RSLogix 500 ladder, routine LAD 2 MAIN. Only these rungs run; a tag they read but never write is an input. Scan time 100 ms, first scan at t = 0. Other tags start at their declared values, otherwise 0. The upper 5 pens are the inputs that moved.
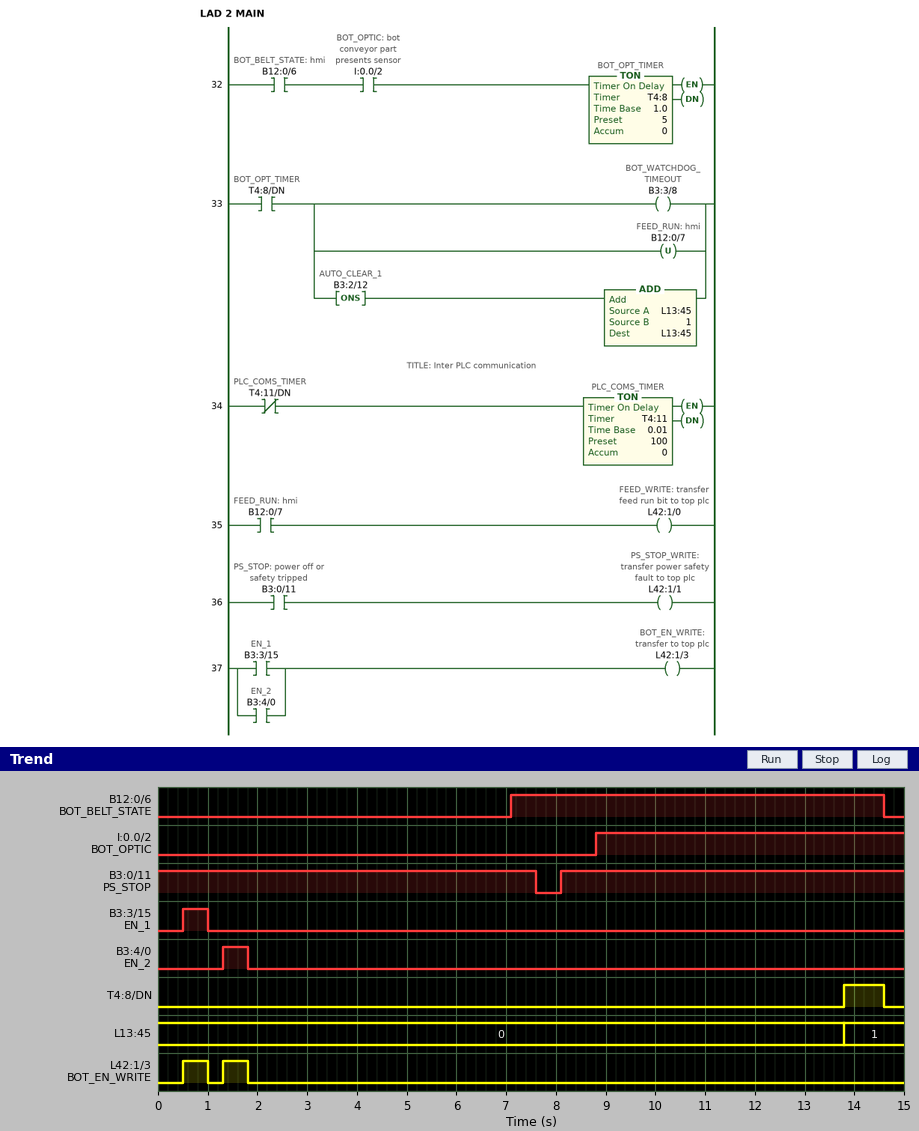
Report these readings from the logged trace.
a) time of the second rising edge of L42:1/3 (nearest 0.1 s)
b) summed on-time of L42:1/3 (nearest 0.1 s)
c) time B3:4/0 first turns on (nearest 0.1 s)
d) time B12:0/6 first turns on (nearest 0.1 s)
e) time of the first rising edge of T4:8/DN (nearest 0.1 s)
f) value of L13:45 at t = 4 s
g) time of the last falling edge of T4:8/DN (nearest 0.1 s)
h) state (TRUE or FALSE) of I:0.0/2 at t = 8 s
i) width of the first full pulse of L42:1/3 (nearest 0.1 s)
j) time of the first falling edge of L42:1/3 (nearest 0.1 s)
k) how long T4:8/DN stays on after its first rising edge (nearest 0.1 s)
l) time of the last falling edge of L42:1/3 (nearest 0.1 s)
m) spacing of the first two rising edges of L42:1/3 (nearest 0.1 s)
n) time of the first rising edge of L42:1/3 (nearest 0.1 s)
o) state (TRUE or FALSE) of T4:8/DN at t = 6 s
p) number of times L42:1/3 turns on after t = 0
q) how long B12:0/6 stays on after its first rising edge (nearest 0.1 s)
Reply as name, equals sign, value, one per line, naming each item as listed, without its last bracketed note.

time of the second rising edge of L42:1/3 = 1.3 s
summed on-time of L42:1/3 = 1.0 s
time B3:4/0 first turns on = 1.3 s
time B12:0/6 first turns on = 7.1 s
time of the first rising edge of T4:8/DN = 13.8 s
value of L13:45 at t = 4 s = 0
time of the last falling edge of T4:8/DN = 14.6 s
state (TRUE or FALSE) of I:0.0/2 at t = 8 s = FALSE
width of the first full pulse of L42:1/3 = 0.5 s
time of the first falling edge of L42:1/3 = 1.0 s
how long T4:8/DN stays on after its first rising edge = 0.8 s
time of the last falling edge of L42:1/3 = 1.8 s
spacing of the first two rising edges of L42:1/3 = 0.8 s
time of the first rising edge of L42:1/3 = 0.5 s
state (TRUE or FALSE) of T4:8/DN at t = 6 s = FALSE
number of times L42:1/3 turns on after t = 0 = 2
how long B12:0/6 stays on after its first rising edge = 7.5 s
